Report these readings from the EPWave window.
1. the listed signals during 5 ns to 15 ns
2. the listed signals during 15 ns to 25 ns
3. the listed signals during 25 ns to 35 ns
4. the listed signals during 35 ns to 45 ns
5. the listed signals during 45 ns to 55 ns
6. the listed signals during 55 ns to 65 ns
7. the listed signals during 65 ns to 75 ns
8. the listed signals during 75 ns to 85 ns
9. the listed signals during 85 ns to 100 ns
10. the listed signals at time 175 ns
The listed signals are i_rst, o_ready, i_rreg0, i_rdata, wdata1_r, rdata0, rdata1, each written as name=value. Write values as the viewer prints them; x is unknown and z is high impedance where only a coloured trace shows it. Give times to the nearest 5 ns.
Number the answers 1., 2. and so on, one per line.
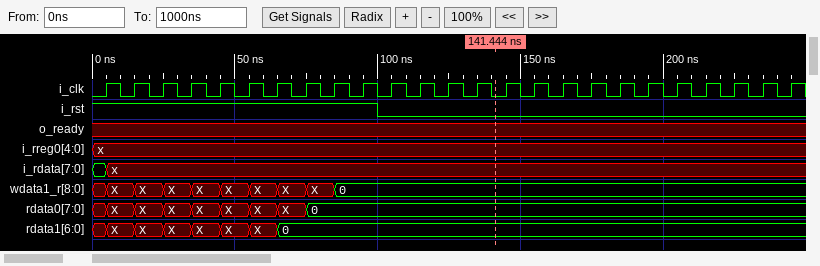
1. i_rst=1, o_ready=x, i_rreg0=x, i_rdata=x, wdata1_r=X, rdata0=X, rdata1=X
2. i_rst=1, o_ready=x, i_rreg0=x, i_rdata=x, wdata1_r=X, rdata0=X, rdata1=X
3. i_rst=1, o_ready=x, i_rreg0=x, i_rdata=x, wdata1_r=X, rdata0=X, rdata1=X
4. i_rst=1, o_ready=x, i_rreg0=x, i_rdata=x, wdata1_r=X, rdata0=X, rdata1=X
5. i_rst=1, o_ready=x, i_rreg0=x, i_rdata=x, wdata1_r=X, rdata0=X, rdata1=X
6. i_rst=1, o_ready=x, i_rreg0=x, i_rdata=x, wdata1_r=X, rdata0=X, rdata1=X
7. i_rst=1, o_ready=x, i_rreg0=x, i_rdata=x, wdata1_r=X, rdata0=X, rdata1=0
8. i_rst=1, o_ready=x, i_rreg0=x, i_rdata=x, wdata1_r=X, rdata0=0, rdata1=0
9. i_rst=1, o_ready=x, i_rreg0=x, i_rdata=x, wdata1_r=0, rdata0=0, rdata1=0
10. i_rst=0, o_ready=x, i_rreg0=x, i_rdata=x, wdata1_r=0, rdata0=0, rdata1=0
